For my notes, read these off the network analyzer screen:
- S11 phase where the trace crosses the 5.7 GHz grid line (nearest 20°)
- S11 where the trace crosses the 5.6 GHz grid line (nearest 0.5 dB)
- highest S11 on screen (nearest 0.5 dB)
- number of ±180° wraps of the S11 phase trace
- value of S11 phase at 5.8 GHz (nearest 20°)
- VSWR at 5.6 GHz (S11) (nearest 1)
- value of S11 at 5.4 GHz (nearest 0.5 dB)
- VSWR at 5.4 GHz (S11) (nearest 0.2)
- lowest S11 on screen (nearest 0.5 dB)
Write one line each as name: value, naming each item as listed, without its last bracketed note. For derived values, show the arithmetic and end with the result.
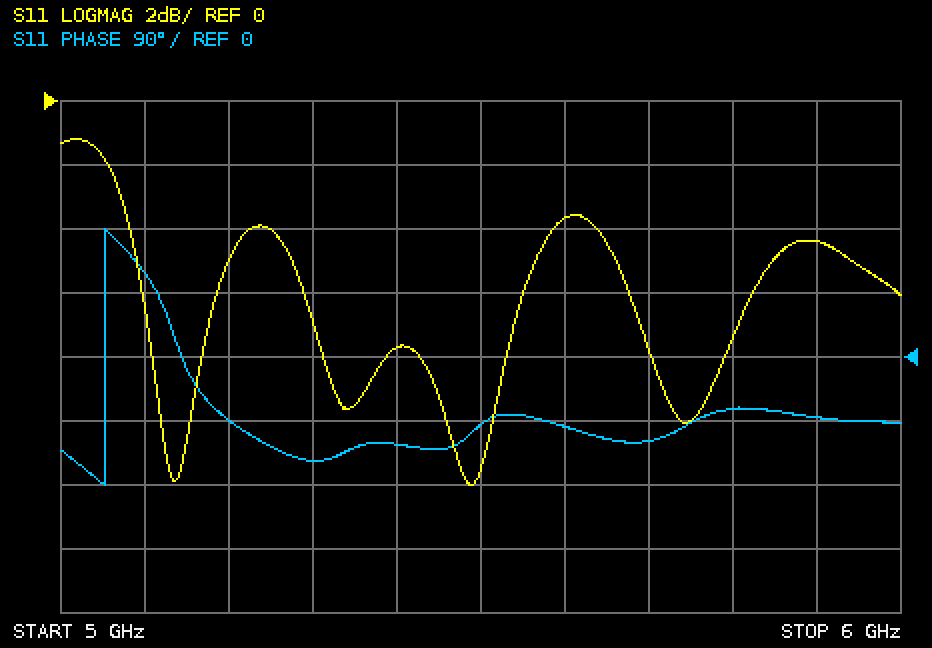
S11 phase where the trace crosses the 5.7 GHz grid line: -120°
S11 where the trace crosses the 5.6 GHz grid line: -3.5 dB
highest S11 on screen: -1.0 dB
number of ±180° wraps of the S11 phase trace: 1
value of S11 phase at 5.8 GHz: -80°
VSWR at 5.6 GHz (S11): |Γ| = 10^(-3.5/20) = 0.6683; VSWR = (1 + 0.6683)/(1 − 0.6683) ≈ 5
value of S11 at 5.4 GHz: -7.5 dB
VSWR at 5.4 GHz (S11): |Γ| = 10^(-7.5/20) = 0.4217; VSWR = (1 + 0.4217)/(1 − 0.4217) ≈ 2.46, so 2.4 to the nearest 0.2
lowest S11 on screen: -12.0 dB
